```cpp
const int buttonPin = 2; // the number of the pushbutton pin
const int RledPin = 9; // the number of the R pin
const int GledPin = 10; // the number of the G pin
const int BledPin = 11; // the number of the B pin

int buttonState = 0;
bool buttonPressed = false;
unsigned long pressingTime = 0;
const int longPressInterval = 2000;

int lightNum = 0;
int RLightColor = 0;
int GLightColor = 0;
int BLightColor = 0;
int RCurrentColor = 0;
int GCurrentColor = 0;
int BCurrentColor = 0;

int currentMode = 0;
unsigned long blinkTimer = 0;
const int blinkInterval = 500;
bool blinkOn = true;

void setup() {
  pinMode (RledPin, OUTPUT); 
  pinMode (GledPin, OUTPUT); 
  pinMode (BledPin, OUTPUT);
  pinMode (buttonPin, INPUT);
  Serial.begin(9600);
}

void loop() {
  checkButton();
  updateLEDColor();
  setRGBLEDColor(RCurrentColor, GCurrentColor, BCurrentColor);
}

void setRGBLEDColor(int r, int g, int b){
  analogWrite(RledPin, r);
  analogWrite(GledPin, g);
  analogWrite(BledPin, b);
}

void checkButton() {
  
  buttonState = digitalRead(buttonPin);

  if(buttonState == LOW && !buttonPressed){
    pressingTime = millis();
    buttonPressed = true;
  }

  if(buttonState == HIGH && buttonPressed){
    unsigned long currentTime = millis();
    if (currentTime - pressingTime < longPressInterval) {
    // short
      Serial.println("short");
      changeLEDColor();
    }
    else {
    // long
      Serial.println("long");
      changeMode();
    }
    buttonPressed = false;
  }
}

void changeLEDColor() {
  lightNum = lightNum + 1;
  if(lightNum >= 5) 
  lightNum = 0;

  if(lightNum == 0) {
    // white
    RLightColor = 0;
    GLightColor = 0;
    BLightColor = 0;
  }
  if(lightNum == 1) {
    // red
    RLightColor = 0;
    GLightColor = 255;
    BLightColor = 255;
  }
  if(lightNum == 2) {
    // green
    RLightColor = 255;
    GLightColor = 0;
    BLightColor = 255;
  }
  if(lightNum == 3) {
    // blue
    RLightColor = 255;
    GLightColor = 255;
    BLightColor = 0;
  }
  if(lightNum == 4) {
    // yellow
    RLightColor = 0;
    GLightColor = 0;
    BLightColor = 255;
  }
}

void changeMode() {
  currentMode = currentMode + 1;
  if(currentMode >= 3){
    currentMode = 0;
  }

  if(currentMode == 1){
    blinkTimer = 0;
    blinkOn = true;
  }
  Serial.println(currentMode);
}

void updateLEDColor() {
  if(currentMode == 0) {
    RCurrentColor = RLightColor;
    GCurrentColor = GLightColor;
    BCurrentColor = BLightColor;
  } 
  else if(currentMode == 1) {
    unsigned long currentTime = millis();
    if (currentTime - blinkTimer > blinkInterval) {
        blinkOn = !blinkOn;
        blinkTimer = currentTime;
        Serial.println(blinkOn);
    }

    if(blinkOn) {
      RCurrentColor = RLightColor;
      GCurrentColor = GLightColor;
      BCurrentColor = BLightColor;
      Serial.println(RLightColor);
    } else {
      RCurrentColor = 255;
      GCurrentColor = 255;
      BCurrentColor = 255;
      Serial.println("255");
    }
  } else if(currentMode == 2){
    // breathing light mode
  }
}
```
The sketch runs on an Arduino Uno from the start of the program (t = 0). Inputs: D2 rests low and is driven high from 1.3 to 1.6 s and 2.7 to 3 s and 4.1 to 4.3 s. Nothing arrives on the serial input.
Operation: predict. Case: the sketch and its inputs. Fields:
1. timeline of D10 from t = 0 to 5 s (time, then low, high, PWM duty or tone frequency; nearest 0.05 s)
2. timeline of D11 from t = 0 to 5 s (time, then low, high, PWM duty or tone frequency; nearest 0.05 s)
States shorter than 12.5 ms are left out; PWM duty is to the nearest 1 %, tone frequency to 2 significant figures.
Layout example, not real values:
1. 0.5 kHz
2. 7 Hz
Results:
1. 0 s low; 1.3 s high; 2.7 s low; 4.1 s high
2. 0 s low; 1.3 s high; 4.1 s low
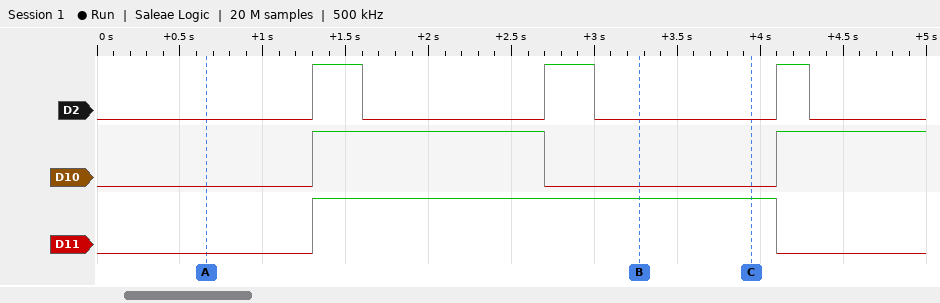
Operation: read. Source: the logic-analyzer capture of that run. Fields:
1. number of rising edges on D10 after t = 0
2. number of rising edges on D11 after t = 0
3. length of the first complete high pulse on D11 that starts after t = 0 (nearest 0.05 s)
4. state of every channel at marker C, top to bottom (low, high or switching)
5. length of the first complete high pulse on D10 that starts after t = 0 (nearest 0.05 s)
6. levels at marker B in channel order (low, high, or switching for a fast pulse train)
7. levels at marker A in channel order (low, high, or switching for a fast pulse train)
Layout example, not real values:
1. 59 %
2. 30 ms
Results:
1. 2
2. 1
3. 2.80 s
4. D2 low, D10 low, D11 high
5. 1.40 s
6. D2 low, D10 low, D11 high
7. D2 low, D10 low, D11 low
